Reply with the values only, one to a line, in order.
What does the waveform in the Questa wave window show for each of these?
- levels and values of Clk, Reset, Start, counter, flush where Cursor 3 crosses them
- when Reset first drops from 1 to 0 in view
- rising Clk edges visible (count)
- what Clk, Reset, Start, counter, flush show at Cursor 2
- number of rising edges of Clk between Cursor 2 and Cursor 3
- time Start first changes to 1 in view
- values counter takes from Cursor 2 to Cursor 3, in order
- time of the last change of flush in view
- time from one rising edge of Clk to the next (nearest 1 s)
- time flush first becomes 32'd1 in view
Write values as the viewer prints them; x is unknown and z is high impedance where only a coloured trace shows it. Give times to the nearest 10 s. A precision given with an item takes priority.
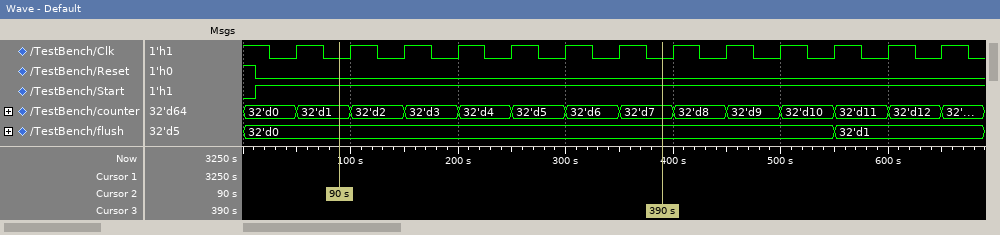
Clk=0, Reset=0, Start=1, counter=32'd7, flush=32'd0
10 s
13
Clk=0, Reset=0, Start=1, counter=32'd1, flush=32'd0
6
10 s
32'd1, 32'd2, 32'd3, 32'd4, 32'd5, 32'd6, 32'd7
550 s
50 s
550 s
